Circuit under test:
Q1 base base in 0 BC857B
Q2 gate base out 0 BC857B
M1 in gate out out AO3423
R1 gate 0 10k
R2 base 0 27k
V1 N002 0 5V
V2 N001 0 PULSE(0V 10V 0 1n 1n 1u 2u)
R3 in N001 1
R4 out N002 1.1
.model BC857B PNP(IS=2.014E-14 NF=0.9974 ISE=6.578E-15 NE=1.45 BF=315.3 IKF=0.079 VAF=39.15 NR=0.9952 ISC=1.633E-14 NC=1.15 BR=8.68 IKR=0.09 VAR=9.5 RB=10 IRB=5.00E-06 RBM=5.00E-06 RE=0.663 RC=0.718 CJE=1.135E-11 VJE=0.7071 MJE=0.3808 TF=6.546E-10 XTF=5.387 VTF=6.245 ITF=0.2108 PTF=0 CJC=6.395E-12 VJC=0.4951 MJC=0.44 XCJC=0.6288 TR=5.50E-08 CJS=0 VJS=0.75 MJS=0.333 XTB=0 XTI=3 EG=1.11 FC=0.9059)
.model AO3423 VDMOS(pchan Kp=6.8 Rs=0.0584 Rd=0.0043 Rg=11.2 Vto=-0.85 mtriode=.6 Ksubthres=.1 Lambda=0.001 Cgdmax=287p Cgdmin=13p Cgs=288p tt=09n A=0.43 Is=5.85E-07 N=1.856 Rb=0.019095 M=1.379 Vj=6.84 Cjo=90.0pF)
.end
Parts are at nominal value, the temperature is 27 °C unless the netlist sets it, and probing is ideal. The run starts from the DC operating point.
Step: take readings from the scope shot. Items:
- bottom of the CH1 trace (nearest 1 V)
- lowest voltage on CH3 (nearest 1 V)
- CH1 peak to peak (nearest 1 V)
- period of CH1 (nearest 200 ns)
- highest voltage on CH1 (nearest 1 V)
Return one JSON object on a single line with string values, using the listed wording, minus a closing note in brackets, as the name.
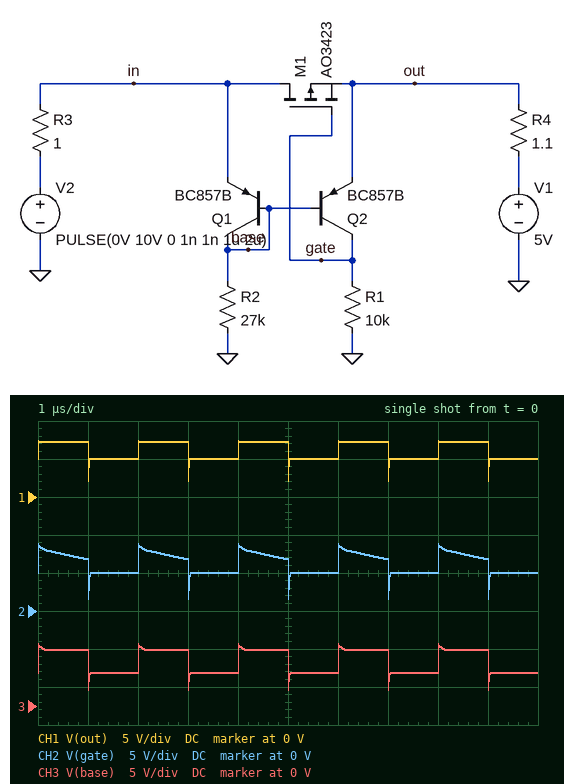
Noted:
{"bottom of the CH1 trace": "2 V", "lowest voltage on CH3": "2 V", "CH1 peak to peak": "5 V", "period of CH1": "2.0 µs", "highest voltage on CH1": "7 V"}
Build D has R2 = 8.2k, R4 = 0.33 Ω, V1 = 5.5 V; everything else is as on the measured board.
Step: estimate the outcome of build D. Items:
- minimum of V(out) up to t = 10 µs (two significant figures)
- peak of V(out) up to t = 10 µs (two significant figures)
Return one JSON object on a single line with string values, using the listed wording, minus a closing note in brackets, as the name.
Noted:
{"minimum of V(out) up to t = 10 µs": "4.0 V", "peak of V(out) up to t = 10 µs": "6.5 V"}
